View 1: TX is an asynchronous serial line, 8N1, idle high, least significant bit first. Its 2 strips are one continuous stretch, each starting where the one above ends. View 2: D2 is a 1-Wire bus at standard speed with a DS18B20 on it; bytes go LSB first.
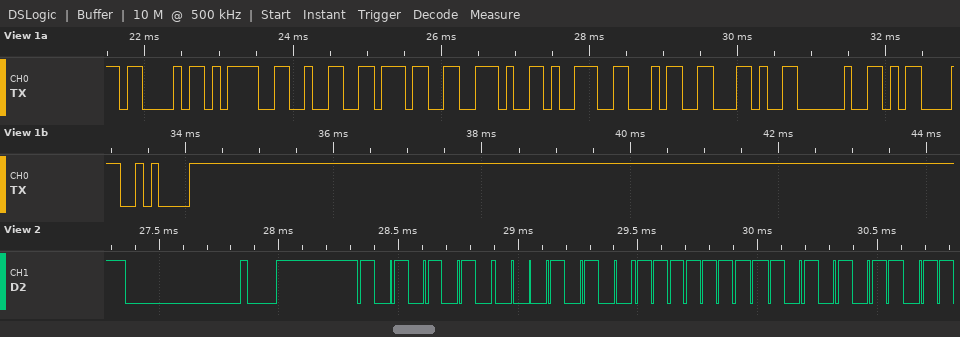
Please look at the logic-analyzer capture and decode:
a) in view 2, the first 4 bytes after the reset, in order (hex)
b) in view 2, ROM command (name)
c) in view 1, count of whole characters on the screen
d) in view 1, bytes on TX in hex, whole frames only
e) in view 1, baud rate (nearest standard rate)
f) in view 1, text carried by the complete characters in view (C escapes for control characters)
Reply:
55 28 FF D5
Match ROM
11
43 3D 32 37 2E 39 34 2C 20 0D 0A
9600 baud
"C=27.94, \r\n"
